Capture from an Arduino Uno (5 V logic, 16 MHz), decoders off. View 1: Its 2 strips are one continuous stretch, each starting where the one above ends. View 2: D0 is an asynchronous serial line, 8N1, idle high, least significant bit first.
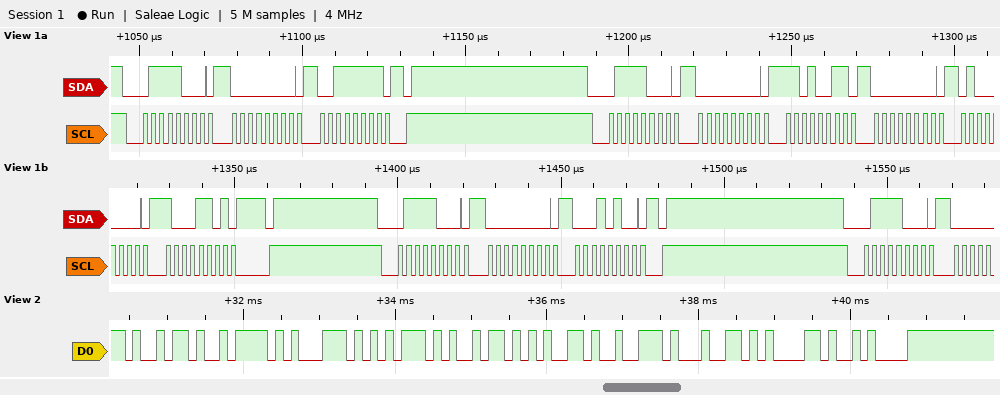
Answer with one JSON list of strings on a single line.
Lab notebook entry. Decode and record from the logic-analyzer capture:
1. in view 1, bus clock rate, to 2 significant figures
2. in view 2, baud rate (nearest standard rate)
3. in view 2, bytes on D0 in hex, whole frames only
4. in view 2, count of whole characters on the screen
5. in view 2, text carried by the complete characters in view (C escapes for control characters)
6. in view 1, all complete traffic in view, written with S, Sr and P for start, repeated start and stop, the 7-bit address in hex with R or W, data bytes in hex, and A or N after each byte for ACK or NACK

["400 kHz", "9600 baud", "69 7A 71 75 69 65 72 64 61 0A", "10", "\"izquierda\\n\"", "S 3CW A 00 A 3F A P S 3CW A 00 A D3 A 00 A 40 A 8D A P S 3CW A 00 A 14 A P S 3CW A"]
